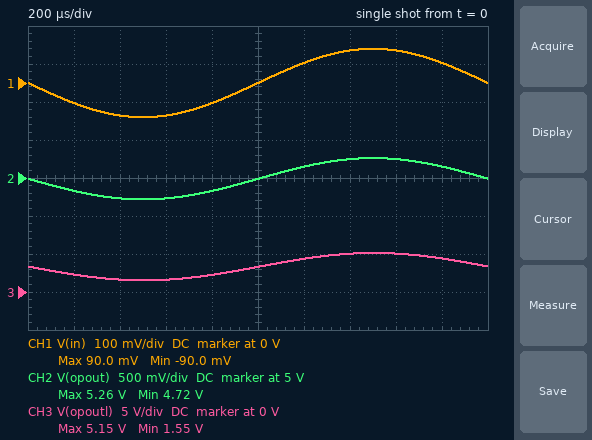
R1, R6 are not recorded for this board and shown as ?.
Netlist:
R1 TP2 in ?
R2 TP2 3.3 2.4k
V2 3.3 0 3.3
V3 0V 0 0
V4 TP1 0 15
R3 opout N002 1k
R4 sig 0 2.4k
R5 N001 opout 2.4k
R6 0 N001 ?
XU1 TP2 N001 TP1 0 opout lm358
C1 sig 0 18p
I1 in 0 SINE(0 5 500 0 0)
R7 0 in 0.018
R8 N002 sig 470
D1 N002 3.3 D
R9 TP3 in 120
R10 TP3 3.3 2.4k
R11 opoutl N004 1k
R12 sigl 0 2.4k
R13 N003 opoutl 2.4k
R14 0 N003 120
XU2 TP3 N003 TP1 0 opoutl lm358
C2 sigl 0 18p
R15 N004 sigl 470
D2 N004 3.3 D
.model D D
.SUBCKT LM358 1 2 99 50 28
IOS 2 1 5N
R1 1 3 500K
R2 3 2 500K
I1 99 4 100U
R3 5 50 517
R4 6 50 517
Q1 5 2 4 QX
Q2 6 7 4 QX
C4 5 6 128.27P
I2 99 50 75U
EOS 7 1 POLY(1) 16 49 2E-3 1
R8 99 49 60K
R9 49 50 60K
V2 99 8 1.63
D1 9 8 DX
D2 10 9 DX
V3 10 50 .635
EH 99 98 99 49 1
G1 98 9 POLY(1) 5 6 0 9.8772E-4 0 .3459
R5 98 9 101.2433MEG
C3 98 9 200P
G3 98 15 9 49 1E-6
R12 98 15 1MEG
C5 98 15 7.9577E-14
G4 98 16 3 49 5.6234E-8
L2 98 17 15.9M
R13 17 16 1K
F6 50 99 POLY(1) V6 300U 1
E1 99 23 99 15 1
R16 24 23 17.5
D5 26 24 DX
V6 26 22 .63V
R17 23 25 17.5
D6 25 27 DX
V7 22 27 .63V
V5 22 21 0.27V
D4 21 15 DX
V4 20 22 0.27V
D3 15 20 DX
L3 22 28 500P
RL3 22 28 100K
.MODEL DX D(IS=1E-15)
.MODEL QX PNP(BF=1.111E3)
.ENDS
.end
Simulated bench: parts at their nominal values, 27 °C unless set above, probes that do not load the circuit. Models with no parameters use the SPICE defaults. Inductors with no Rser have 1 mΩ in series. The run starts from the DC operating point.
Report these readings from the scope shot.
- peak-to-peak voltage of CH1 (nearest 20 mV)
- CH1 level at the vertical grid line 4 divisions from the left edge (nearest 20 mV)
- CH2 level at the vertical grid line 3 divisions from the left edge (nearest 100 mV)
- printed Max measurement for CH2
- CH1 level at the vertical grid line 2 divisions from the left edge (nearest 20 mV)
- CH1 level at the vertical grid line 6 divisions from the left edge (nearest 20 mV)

180 mV
-60 mV
4.7 V
5.26 V
-80 mV
60 mV
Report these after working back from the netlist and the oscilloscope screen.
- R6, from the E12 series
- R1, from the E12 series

680 Ω
1.2 kΩ
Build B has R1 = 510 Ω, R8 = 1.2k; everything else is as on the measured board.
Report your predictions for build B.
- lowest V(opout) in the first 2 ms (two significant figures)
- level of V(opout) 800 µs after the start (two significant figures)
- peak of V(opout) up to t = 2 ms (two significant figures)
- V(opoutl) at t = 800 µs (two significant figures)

2.3 V
2.4 V
3.0 V
2.3 V
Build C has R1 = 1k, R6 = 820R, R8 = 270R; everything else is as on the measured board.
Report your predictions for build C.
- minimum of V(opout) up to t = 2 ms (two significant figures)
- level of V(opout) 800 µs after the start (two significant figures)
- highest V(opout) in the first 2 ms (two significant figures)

3.6 V
3.7 V
4.1 V
